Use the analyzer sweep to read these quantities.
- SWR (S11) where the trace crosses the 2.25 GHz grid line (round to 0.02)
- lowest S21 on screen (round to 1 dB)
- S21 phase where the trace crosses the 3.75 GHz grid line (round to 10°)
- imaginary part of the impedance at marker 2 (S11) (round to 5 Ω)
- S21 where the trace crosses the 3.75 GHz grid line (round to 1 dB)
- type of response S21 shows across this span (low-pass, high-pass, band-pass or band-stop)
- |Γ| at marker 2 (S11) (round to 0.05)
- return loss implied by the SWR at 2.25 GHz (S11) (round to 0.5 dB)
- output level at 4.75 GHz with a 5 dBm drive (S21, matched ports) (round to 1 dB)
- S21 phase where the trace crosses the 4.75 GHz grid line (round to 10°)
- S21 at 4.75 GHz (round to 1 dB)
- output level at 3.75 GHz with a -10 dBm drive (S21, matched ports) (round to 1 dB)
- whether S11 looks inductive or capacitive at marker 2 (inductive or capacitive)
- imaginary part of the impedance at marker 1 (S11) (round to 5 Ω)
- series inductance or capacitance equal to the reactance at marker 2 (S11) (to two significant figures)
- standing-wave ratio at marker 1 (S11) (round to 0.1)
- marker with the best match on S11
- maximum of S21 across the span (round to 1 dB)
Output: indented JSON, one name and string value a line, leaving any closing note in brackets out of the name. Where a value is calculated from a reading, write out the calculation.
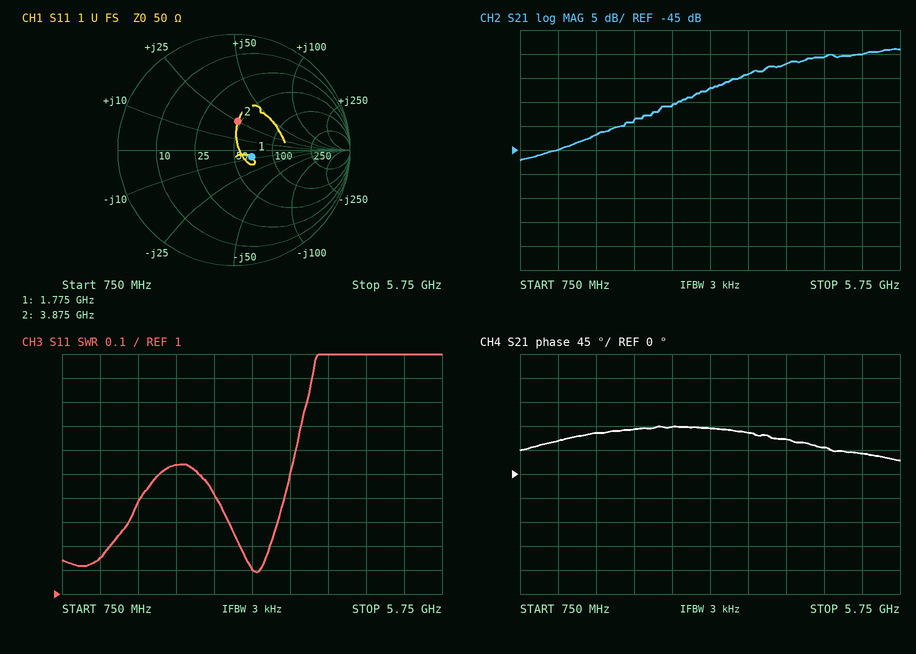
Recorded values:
{
  "SWR (S11) where the trace crosses the 2.25 GHz grid line": "1.54",
  "lowest S21 on screen": "-47 dB",
  "S21 phase where the trace crosses the 3.75 GHz grid line": "80°",
  "imaginary part of the impedance at marker 2 (S11)": "+25 Ω",
  "S21 where the trace crosses the 3.75 GHz grid line": "-29 dB",
  "type of response S21 shows across this span": "high-pass",
  "|Γ| at marker 2 (S11)": "0.25",
  "return loss implied by the SWR at 2.25 GHz (S11)": "−20 log10((1.54 − 1)/(1.54 + 1)) ≈ 13.4 dB, so 13.5 dB to the nearest 0.5 dB",
  "output level at 4.75 GHz with a 5 dBm drive (S21, matched ports)": "5 dBm + (-26 dB) = -21 dBm",
  "S21 phase where the trace crosses the 4.75 GHz grid line": "50°",
  "S21 at 4.75 GHz": "-26 dB",
  "output level at 3.75 GHz with a -10 dBm drive (S21, matched ports)": "-10 dBm + (-29 dB) = -39 dBm",
  "whether S11 looks inductive or capacitive at marker 2": "inductive",
  "imaginary part of the impedance at marker 1 (S11)": "-10 Ω",
  "series inductance or capacitance equal to the reactance at marker 2 (S11)": "L = 25 Ω/(2π × 3.875 GHz) ≈ 1.0 nH",
  "standing-wave ratio at marker 1 (S11)": "1.4",
  "marker with the best match on S11": "marker 1",
  "maximum of S21 across the span": "-24 dB"
}
